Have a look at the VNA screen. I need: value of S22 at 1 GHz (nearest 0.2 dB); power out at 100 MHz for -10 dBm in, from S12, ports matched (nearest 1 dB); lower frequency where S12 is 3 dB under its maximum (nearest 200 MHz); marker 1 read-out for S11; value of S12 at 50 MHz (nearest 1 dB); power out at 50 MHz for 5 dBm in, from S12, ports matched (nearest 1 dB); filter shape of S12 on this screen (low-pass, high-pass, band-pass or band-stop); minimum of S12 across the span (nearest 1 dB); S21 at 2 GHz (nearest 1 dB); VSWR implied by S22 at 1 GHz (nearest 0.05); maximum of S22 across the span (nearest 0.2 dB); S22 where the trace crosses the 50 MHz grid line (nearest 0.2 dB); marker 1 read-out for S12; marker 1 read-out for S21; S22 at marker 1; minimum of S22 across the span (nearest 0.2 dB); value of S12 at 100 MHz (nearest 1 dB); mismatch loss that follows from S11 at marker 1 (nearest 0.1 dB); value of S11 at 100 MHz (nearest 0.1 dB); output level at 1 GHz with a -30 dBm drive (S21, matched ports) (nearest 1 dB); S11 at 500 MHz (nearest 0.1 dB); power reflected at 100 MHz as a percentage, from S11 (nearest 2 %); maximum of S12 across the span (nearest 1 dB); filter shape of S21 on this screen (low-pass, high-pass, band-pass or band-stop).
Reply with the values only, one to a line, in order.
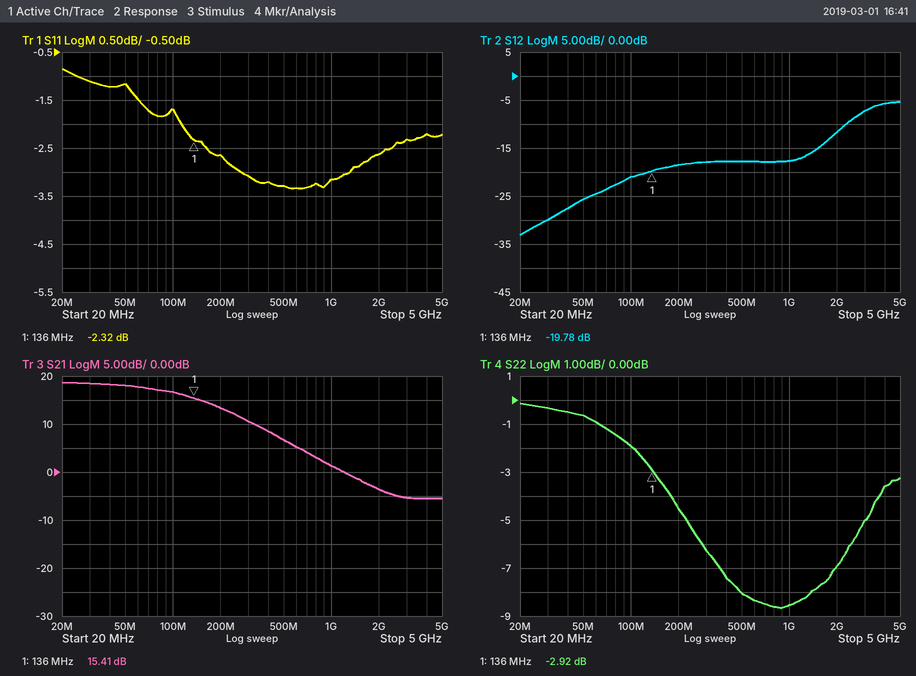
-8.6 dB
-31 dBm
2.6 GHz
-2.32 dB
-26 dB
-21 dBm
high-pass
-33 dB
-4 dB
2.20
-0.2 dB
-0.6 dB
-19.78 dB
15.41 dB
-2.92 dB
-8.6 dB
-21 dB
3.8 dB
-1.7 dB
-29 dBm
-3.3 dB
68 %
-5 dB
low-pass
